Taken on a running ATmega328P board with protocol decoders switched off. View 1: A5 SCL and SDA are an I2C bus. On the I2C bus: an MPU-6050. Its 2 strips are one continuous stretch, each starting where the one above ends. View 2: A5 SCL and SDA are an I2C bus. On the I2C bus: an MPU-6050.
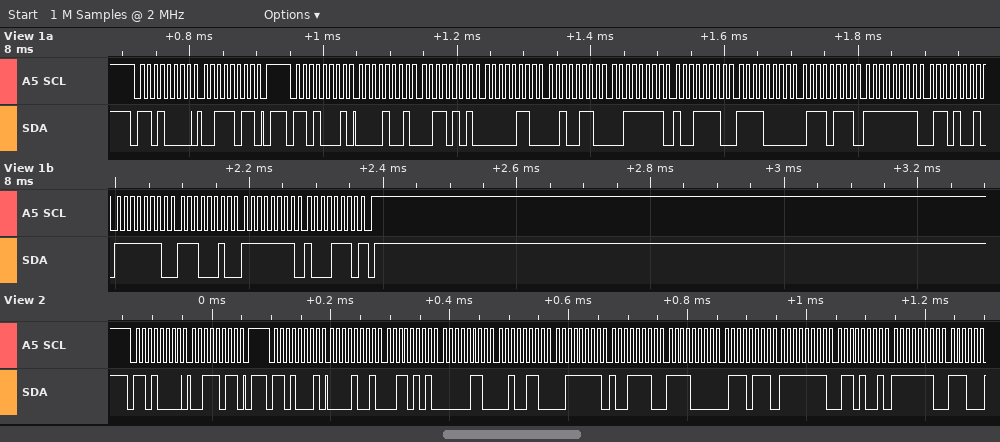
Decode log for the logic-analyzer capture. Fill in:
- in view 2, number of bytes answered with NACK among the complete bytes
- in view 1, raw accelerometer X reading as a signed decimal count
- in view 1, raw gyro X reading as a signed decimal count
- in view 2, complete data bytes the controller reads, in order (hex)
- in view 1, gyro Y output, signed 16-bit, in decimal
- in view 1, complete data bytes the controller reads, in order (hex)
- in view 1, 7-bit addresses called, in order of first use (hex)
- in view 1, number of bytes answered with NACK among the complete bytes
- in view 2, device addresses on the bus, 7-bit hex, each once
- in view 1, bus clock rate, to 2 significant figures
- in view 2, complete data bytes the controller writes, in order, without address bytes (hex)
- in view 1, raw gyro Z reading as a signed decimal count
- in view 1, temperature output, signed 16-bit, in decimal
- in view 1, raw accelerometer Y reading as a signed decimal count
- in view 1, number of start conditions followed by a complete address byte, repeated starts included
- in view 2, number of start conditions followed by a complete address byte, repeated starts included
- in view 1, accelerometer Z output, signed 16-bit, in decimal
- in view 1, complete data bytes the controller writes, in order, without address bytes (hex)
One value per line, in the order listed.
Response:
0
2357
-151
09 35 06 26 3F 9E F0 77 FF 69 FE
-286
09 35 06 26 3F 9E F0 77 FF 69 FE E2 FF 8E
0x68
1
0x68
100 kHz
3B
-114
-3977
1574
2
2
16286
3B
